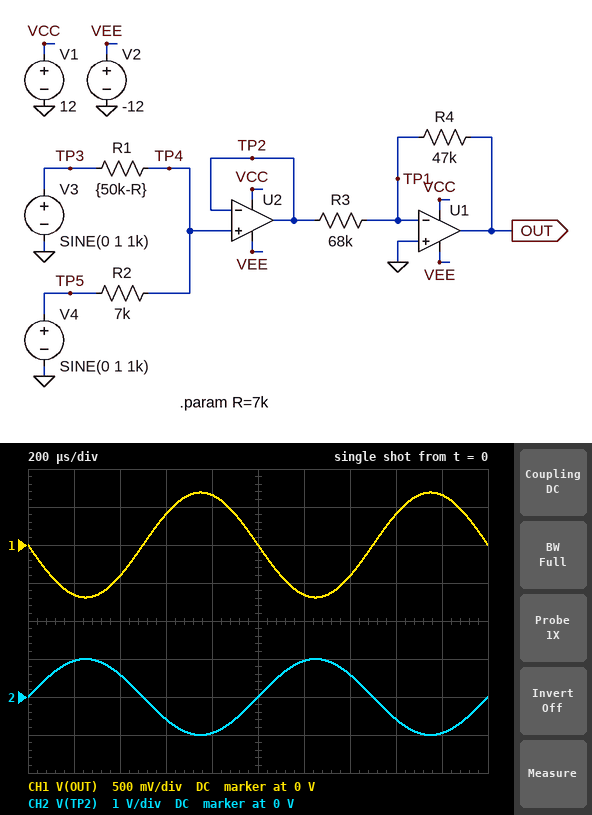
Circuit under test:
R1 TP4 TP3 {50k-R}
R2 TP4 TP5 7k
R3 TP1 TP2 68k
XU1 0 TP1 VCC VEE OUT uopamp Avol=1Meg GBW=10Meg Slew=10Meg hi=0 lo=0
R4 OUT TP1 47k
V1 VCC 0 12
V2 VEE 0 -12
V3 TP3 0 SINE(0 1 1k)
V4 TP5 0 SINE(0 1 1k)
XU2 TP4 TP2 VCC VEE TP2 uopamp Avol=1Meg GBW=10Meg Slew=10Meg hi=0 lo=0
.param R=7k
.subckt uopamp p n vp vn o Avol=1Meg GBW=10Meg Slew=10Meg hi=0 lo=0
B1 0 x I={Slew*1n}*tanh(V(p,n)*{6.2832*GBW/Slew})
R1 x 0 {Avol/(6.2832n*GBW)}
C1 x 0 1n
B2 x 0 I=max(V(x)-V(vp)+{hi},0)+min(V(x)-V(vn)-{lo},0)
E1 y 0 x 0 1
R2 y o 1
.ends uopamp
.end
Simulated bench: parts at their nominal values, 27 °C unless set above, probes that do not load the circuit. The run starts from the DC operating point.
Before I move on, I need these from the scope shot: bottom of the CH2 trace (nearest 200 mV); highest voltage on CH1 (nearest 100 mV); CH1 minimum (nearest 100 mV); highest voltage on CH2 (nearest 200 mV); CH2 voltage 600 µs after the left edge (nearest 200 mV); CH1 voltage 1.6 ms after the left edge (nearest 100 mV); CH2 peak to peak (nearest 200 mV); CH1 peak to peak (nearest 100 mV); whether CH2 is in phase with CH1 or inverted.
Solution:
-1.0 V
700 mV
-700 mV
1.0 V
-600 mV
400 mV
2.0 V
1.4 V
inverted
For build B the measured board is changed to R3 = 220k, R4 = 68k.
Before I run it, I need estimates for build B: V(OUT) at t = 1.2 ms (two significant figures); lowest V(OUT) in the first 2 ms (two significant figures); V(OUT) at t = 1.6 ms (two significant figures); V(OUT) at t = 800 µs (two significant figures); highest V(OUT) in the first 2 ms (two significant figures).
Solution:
-290 mV
-310 mV
180 mV
290 mV
310 mV
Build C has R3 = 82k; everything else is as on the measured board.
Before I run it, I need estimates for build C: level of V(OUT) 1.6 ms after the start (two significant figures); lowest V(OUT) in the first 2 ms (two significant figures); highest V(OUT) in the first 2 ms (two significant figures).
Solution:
340 mV
-570 mV
570 mV
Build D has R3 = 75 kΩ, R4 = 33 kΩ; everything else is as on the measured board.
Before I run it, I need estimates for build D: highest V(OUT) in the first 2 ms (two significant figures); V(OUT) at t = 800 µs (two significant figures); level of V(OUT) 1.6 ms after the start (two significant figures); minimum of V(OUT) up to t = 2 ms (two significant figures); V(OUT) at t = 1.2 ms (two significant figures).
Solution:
440 mV
420 mV
260 mV
-440 mV
-420 mV
